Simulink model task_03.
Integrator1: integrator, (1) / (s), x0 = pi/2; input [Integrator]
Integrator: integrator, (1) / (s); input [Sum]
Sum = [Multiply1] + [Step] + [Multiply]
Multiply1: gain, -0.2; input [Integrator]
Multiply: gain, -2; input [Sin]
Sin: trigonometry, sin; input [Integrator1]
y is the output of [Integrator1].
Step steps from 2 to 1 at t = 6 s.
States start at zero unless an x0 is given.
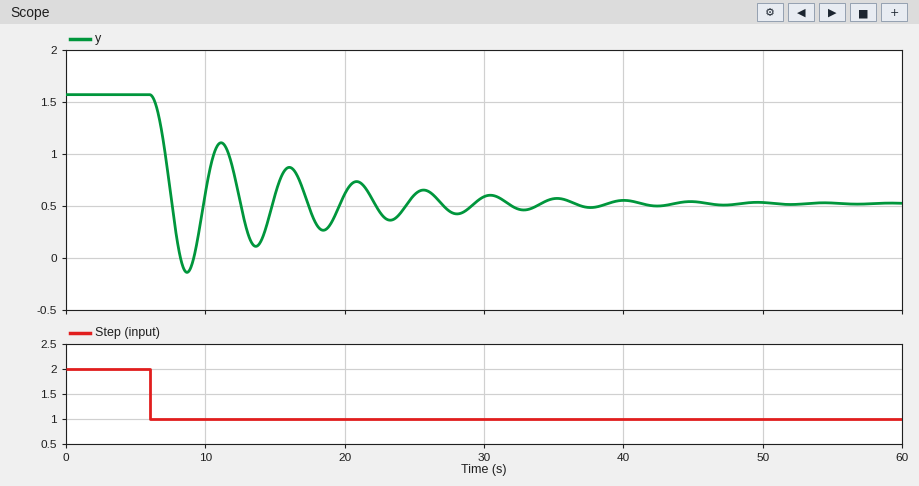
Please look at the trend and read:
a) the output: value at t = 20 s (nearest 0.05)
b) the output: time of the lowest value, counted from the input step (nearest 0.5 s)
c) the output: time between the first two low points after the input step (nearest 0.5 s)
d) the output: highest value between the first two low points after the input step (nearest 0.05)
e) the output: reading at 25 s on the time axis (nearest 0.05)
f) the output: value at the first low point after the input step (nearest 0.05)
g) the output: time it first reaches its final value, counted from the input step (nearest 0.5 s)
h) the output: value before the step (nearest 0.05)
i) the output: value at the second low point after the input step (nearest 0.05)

0.60
2.5 s
5.0 s
1.10
0.60
-0.15
1.5 s
1.55
0.10
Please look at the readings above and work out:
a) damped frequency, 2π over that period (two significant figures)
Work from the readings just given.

1.3 rad/s
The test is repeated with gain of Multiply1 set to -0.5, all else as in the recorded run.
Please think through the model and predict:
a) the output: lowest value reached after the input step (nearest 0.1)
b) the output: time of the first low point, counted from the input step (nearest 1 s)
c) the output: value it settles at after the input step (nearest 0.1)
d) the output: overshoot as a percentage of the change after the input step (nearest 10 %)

0.1
3 s
0.5
40 %
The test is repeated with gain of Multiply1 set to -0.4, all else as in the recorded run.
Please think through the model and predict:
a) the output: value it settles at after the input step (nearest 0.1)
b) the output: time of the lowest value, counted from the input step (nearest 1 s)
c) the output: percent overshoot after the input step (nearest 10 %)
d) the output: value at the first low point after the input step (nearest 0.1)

0.5
3 s
50 %
0.0
